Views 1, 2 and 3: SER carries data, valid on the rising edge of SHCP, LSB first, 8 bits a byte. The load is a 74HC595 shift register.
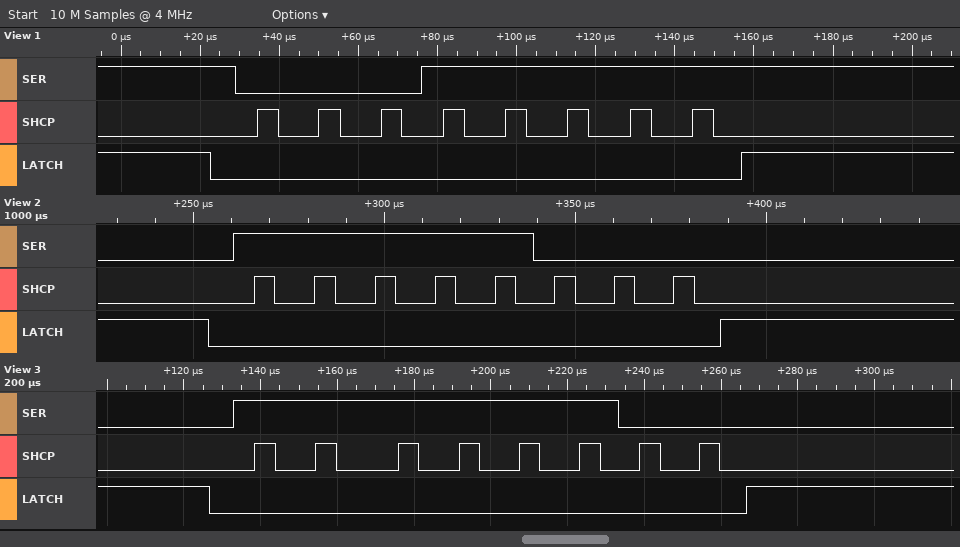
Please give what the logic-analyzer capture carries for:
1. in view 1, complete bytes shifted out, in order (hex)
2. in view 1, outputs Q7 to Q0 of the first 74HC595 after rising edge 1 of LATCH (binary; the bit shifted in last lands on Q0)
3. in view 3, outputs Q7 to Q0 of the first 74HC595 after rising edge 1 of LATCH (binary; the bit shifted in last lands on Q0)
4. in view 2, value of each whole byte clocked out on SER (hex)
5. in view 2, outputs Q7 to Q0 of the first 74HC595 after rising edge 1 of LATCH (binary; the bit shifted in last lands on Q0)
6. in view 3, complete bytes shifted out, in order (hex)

F8
00011111
11111100
1F
11111000
3F
